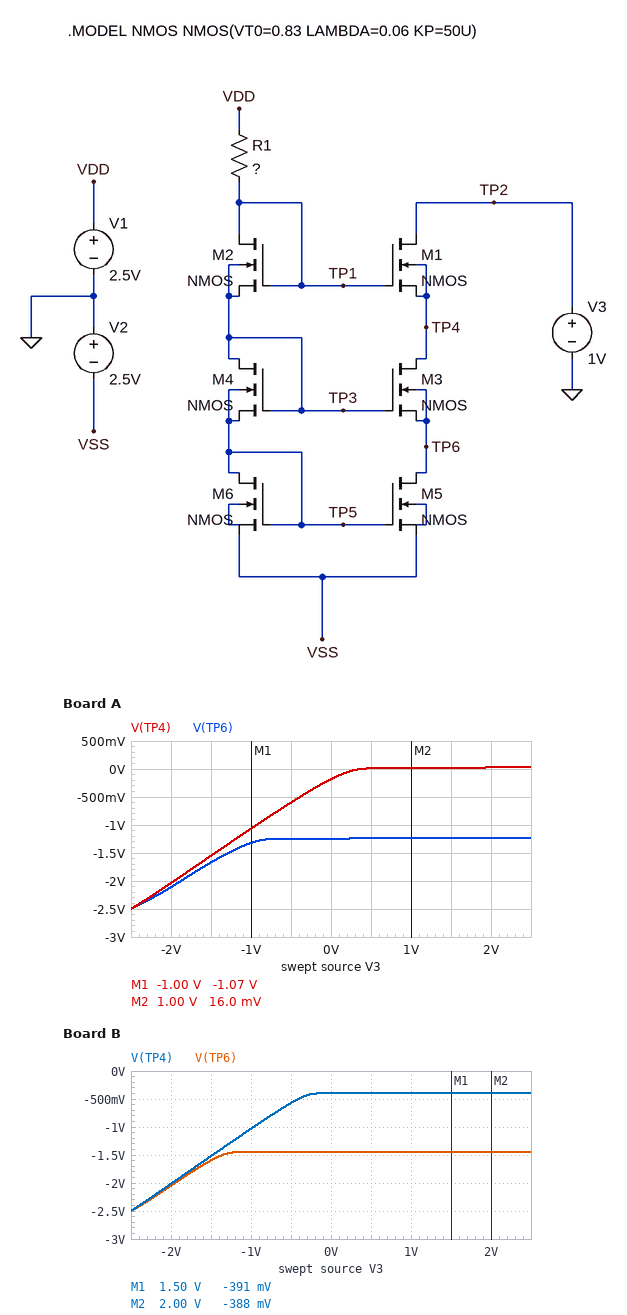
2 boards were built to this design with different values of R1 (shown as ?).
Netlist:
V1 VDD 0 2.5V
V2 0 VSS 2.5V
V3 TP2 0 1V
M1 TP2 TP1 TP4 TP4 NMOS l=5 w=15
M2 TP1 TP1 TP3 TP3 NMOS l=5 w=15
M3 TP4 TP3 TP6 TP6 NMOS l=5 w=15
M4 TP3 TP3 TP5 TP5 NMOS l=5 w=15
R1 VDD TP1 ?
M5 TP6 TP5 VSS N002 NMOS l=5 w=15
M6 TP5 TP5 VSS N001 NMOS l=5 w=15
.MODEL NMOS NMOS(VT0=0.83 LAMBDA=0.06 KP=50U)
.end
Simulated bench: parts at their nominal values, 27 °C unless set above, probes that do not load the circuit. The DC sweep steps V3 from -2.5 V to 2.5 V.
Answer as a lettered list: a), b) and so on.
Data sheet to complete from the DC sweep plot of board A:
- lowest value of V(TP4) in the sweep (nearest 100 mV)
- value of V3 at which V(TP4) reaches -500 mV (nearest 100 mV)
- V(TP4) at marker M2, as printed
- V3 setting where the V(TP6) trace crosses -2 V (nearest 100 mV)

a) -2.5 V
b) -400 mV
c) 16.0 mV
d) -1.9 V
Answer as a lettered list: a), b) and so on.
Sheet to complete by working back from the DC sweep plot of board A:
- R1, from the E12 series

a) 82 kΩ
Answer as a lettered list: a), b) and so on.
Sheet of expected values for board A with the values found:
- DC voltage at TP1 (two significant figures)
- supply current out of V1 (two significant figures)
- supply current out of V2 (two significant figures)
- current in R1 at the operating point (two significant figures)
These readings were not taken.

a) 1.3 V
b) 15 µA
c) 30 µA
d) 15 µA
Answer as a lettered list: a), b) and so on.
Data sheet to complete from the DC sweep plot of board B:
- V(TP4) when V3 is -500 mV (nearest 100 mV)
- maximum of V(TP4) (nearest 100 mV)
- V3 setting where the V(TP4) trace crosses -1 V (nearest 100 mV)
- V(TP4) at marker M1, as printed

a) -600 mV
b) -400 mV
c) -1.0 V
d) -391 mV
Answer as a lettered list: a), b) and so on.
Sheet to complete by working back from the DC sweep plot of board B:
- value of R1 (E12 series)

a) 470 kΩ
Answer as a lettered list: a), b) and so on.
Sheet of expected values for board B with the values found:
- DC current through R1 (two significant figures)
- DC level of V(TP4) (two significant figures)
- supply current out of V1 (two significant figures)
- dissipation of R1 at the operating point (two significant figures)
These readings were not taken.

a) 3.9 µA
b) -390 mV
c) 3.9 µA
d) 7.2 µW
